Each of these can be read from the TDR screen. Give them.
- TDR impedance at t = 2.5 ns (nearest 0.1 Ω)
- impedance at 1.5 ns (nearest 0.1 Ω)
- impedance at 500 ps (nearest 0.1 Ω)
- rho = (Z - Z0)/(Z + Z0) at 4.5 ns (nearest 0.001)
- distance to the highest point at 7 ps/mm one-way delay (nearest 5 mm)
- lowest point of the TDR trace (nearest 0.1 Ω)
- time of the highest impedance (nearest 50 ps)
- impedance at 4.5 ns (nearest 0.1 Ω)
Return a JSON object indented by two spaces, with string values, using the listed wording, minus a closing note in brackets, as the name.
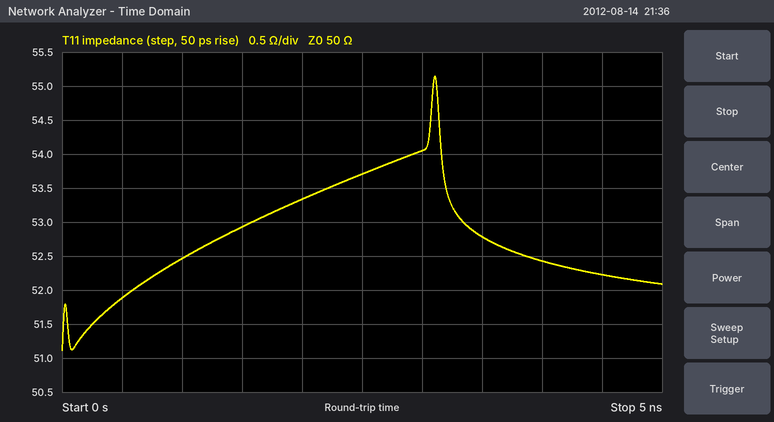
{
  "TDR impedance at t = 2.5 ns": "53.7 Ω",
  "impedance at 1.5 ns": "52.9 Ω",
  "impedance at 500 ps": "51.9 Ω",
  "rho = (Z - Z0)/(Z + Z0) at 4.5 ns": "+0.022",
  "distance to the highest point at 7 ps/mm one-way delay": "220 mm",
  "lowest point of the TDR trace": "51.1 Ω",
  "time of the highest impedance": "3.10 ns",
  "impedance at 4.5 ns": "52.2 Ω"
}
